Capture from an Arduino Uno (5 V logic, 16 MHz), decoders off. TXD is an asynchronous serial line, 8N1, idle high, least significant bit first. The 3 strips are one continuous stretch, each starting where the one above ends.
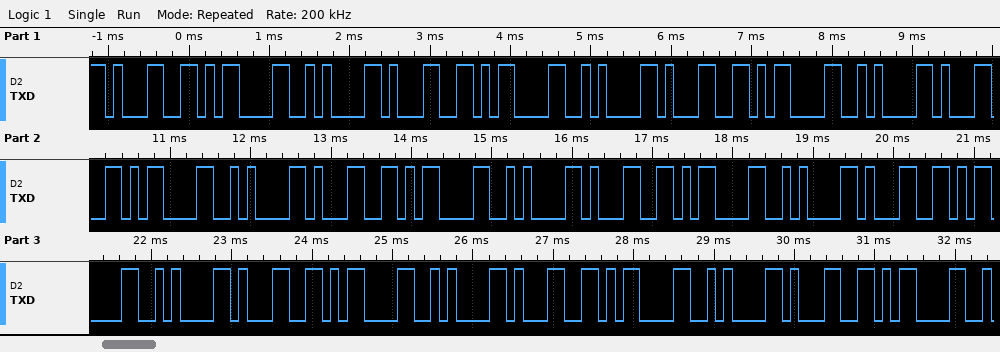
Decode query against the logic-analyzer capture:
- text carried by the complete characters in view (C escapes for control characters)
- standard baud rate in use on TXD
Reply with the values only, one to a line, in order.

"1\r\n1\r\n1\r\n1\r\n1\r\n1\r\n1\r\n1\r\n1\r\n1\r"
9600 baud
